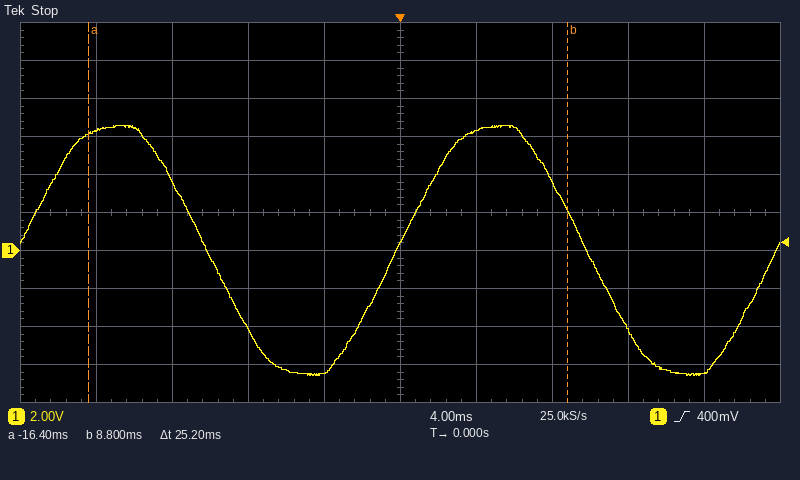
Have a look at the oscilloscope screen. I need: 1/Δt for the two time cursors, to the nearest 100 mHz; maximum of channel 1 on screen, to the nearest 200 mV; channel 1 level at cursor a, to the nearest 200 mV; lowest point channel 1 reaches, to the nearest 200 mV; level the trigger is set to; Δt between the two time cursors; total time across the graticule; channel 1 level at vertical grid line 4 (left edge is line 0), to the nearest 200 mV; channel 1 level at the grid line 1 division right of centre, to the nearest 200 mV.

39.7 Hz
6.6 V
6.2 V
-6.6 V
400 mV
25.2 ms
40 ms
-6.4 V
6.2 V
